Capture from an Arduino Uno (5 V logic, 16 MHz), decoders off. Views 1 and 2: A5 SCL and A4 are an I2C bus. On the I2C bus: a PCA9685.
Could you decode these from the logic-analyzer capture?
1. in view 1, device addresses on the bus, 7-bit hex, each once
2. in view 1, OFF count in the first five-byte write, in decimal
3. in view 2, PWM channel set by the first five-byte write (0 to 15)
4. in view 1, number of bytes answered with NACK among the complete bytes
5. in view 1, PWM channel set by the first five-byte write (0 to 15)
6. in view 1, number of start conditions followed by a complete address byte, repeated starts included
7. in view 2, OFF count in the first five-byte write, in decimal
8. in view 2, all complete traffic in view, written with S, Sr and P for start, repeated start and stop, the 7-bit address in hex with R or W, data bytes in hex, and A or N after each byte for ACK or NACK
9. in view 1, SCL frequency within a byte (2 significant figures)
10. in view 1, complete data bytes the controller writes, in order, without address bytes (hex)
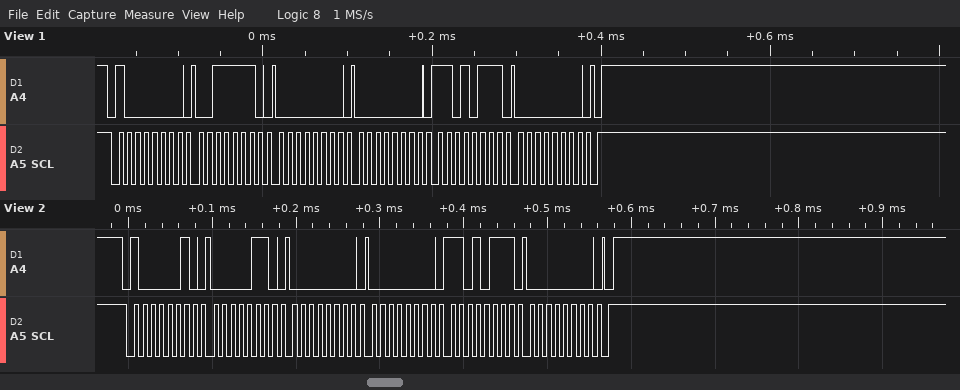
0x40
215
0
0
14
1
215
S 41W A 06 A 00 A 00 A D7 A 00 A P
100 kHz
3E 00 00 D7 00
